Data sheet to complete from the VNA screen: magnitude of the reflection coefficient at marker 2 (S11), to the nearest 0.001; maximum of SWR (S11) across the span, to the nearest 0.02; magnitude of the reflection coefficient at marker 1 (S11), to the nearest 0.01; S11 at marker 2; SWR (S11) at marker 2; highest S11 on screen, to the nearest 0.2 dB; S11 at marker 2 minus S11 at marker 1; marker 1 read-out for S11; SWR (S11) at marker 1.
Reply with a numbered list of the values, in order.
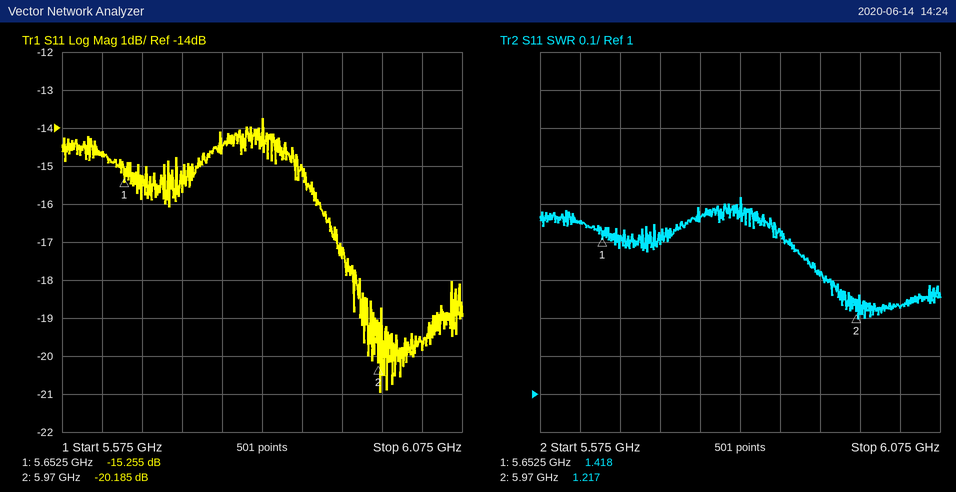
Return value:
1. 0.098
2. 1.52
3. 0.17
4. -20.185 dB
5. 1.217
6. -13.8 dB
7. -4.930 dB
8. -15.255 dB
9. 1.418
